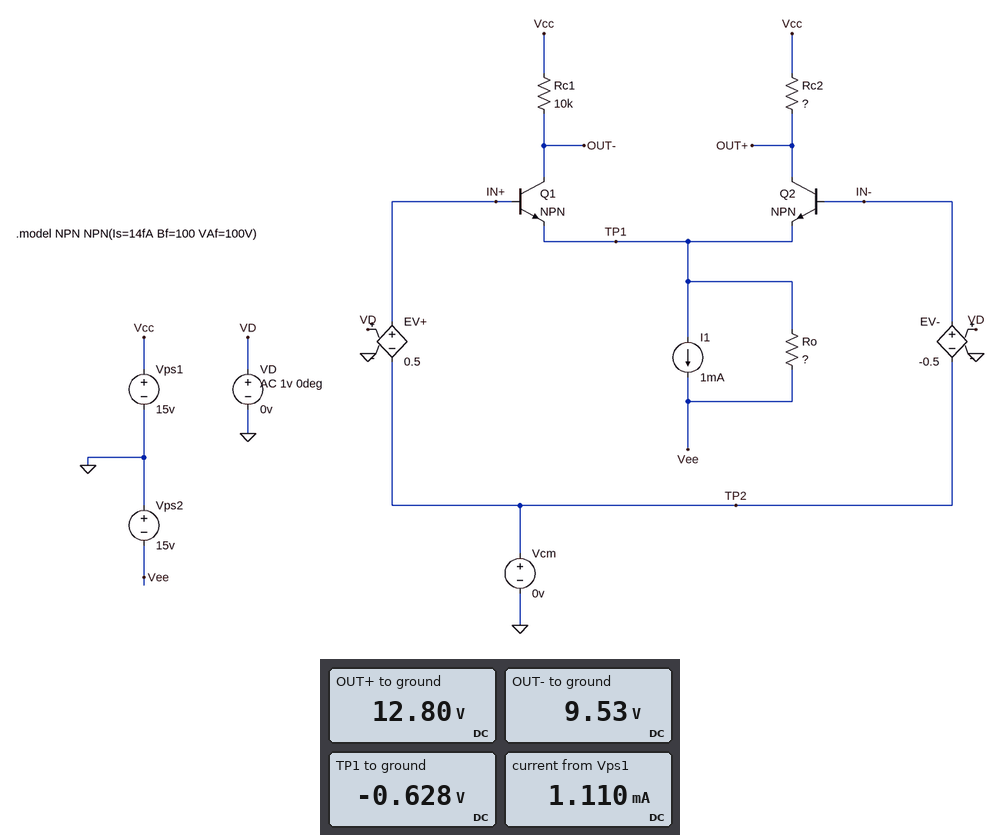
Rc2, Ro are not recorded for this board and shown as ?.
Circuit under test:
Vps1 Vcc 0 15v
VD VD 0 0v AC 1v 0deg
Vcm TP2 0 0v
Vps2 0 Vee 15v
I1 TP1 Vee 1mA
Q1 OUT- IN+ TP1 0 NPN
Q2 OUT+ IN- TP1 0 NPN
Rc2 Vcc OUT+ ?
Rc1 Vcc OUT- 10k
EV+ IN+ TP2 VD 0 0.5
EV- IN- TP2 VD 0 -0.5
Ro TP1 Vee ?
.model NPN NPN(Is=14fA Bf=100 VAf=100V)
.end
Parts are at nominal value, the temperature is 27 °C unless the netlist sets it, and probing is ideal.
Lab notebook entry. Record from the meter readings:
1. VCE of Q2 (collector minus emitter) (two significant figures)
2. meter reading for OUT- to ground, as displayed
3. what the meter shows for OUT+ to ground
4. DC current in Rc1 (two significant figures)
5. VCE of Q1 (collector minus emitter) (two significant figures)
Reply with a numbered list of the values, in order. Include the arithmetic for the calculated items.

1. 12.8 V - (-628 mV) = 13 V
2. 9.53 V
3. 12.80 V
4. (15 V - 9.53 V) / 10 kΩ = 550 µA
5. 9.53 V - (-628 mV) = 10 V
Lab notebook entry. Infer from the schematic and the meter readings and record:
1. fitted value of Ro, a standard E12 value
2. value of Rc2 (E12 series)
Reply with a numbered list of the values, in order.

1. 120 kΩ
2. 3.9 kΩ
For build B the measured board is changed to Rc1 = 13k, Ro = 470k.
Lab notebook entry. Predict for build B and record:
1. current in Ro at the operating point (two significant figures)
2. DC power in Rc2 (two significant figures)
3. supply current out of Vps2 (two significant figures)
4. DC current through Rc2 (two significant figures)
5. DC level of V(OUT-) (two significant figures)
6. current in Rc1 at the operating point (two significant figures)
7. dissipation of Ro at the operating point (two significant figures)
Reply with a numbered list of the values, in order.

1. 31 µA
2. 1.1 mW
3. 1.0 mA
4. 520 µA
5. 8.5 V
6. 500 µA
7. 440 µW
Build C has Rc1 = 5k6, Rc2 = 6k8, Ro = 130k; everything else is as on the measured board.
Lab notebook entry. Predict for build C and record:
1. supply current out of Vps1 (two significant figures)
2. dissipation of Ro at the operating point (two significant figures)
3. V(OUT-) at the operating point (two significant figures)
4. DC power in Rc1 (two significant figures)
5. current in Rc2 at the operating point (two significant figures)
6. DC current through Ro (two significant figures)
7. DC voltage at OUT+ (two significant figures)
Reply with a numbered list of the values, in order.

1. 1.1 mA
2. 1.6 mW
3. 12 V
4. 1.7 mW
5. 550 µA
6. 110 µA
7. 11 V
